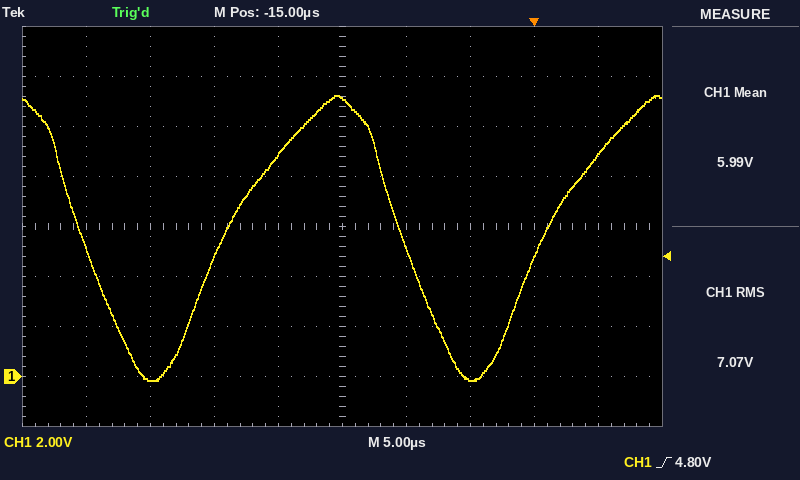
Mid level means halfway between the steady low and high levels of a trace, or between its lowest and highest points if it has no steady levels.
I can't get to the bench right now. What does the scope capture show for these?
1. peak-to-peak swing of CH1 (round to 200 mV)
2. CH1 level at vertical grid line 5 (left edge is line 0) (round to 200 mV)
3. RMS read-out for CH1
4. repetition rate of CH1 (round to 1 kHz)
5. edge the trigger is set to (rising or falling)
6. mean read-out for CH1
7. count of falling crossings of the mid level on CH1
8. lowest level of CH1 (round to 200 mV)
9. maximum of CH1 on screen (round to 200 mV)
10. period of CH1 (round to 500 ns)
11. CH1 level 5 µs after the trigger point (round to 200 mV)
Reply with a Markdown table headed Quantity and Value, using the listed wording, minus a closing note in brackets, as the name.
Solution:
| Quantity | Value |
|---|---|
| peak-to-peak swing of CH1 | 11.4 V |
| CH1 level at vertical grid line 5 (left edge is line 0) | 11.2 V |
| RMS read-out for CH1 | 7.07 V |
| repetition rate of CH1 | 40 kHz |
| edge the trigger is set to | rising |
| mean read-out for CH1 | 5.99 V |
| count of falling crossings of the mid level on CH1 | 2 |
| lowest level of CH1 | -200 mV |
| maximum of CH1 on screen | 11.2 V |
| period of CH1 | 25.0 µs |
| CH1 level 5 µs after the trigger point | 8.8 V |
